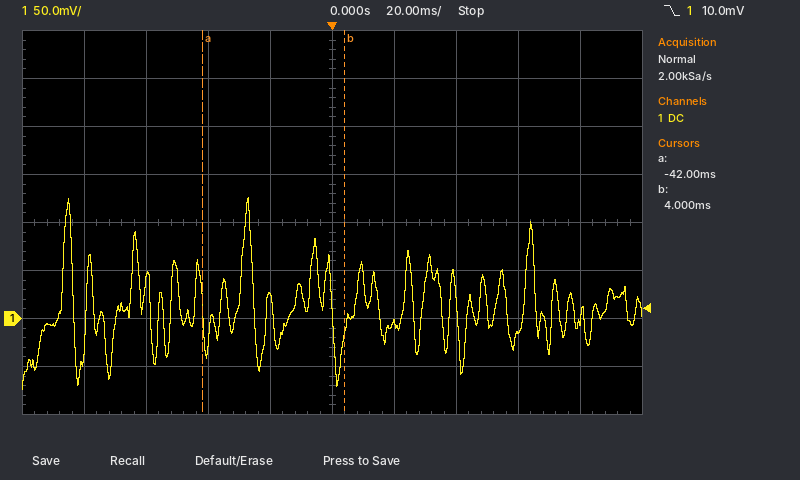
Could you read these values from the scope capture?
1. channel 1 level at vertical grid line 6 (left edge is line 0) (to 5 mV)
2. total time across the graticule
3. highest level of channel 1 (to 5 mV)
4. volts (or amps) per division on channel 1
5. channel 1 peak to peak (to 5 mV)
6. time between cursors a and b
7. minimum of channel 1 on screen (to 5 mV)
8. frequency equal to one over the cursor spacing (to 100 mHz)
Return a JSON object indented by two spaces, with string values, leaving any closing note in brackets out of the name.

{
  "channel 1 level at vertical grid line 6 (left edge is line 0)": "-5 mV",
  "total time across the graticule": "200 ms",
  "highest level of channel 1": "125 mV",
  "volts (or amps) per division on channel 1": "50 mV",
  "channel 1 peak to peak": "200 mV",
  "time between cursors a and b": "46 ms",
  "minimum of channel 1 on screen": "-75 mV",
  "frequency equal to one over the cursor spacing": "21.7 Hz"
}
